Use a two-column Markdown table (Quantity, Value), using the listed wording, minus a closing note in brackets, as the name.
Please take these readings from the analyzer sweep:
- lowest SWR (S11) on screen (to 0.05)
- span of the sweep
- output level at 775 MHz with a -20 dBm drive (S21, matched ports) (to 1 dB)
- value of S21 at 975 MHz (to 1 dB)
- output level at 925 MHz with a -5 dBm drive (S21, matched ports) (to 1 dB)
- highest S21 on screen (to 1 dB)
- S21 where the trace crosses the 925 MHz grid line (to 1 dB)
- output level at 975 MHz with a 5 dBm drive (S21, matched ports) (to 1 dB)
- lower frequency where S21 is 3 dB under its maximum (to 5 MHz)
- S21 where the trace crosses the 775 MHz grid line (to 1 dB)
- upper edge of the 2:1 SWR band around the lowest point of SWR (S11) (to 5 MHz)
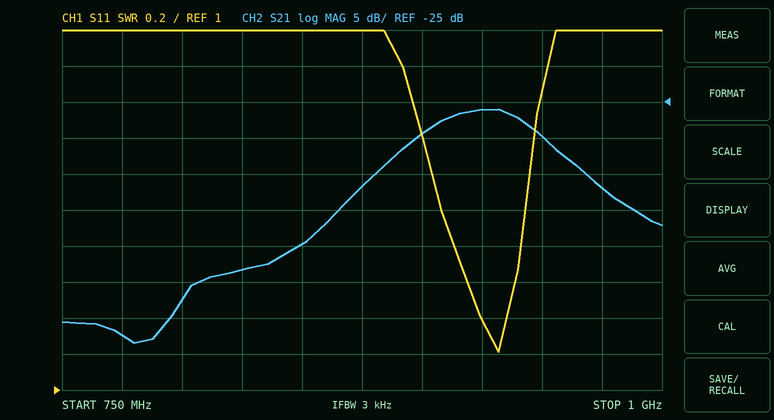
| Quantity | Value |
|---|---|
| lowest SWR (S11) on screen | 1.20 |
| span of the sweep | 250 MHz |
| output level at 775 MHz with a -20 dBm drive (S21, matched ports) | -77 dBm |
| value of S21 at 975 MHz | -37 dB |
| output level at 925 MHz with a -5 dBm drive (S21, matched ports) | -31 dBm |
| highest S21 on screen | -26 dB |
| S21 where the trace crosses the 925 MHz grid line | -26 dB |
| output level at 975 MHz with a 5 dBm drive (S21, matched ports) | -32 dBm |
| lower frequency where S21 is 3 dB under its maximum | 900 MHz |
| S21 where the trace crosses the 775 MHz grid line | -57 dB |
| upper edge of the 2:1 SWR band around the lowest point of SWR (S11) | 945 MHz |
